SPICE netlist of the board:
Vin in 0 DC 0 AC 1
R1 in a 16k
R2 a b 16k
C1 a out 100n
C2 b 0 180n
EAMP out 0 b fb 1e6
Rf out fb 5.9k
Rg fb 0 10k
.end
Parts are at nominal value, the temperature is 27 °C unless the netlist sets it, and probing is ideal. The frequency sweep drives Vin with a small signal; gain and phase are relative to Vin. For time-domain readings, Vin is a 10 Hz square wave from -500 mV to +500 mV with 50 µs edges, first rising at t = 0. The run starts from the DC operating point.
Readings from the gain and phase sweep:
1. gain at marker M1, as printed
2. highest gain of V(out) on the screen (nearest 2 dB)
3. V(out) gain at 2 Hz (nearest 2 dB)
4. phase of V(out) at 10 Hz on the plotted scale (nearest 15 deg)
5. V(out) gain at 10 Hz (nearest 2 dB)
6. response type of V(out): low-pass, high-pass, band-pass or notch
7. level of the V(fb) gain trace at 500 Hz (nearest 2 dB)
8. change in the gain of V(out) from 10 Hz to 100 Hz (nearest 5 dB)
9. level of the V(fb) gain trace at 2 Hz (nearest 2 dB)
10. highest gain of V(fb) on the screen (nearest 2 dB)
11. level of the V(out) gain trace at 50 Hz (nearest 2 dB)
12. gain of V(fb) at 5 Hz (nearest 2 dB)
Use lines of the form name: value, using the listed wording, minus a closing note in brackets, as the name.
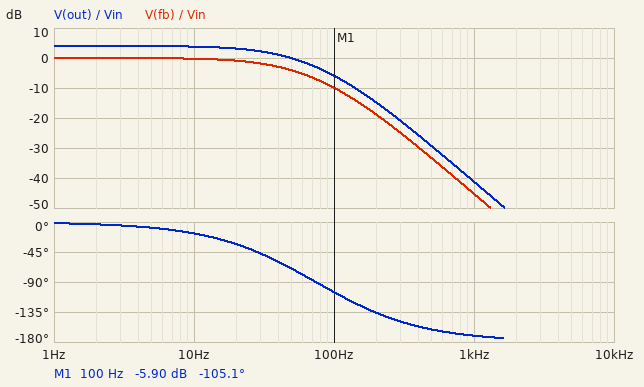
gain at marker M1, as printed: -5.90 dB
highest gain of V(out) on the screen: 4 dB
V(out) gain at 2 Hz: 4 dB
phase of V(out) at 10 Hz on the plotted scale: -15 deg
V(out) gain at 10 Hz: 4 dB
response type of V(out): low-pass, high-pass, band-pass or notch: low-pass
level of the V(fb) gain trace at 500 Hz: -34 dB
change in the gain of V(out) from 10 Hz to 100 Hz: -10 dB
level of the V(fb) gain trace at 2 Hz: 0 dB
highest gain of V(fb) on the screen: 0 dB
level of the V(out) gain trace at 50 Hz: 0 dB
gain of V(fb) at 5 Hz: 0 dB
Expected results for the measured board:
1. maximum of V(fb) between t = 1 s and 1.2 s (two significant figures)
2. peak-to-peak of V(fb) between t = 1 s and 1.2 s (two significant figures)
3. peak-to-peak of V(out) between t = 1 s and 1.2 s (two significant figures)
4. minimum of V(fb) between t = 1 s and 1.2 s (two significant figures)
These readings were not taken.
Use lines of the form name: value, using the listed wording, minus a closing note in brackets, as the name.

maximum of V(fb) between t = 1 s and 1.2 s: 500 mV
peak-to-peak of V(fb) between t = 1 s and 1.2 s: 1.0 V
peak-to-peak of V(out) between t = 1 s and 1.2 s: 1.6 V
minimum of V(fb) between t = 1 s and 1.2 s: -500 mV
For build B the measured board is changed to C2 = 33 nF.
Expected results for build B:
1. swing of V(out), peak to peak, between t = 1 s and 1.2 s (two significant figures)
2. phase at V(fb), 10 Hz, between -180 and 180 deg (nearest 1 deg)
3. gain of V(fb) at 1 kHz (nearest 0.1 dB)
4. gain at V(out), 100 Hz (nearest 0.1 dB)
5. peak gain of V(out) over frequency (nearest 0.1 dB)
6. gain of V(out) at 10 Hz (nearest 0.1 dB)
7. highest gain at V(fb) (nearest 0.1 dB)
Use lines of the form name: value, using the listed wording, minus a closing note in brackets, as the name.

swing of V(out), peak to peak, between t = 1 s and 1.2 s: 4.3 V
phase at V(fb), 10 Hz, between -180 and 180 deg: 0 deg
gain of V(fb) at 1 kHz: -30.2 dB
gain at V(out), 100 Hz: 7.5 dB
peak gain of V(out) over frequency: 22.3 dB
gain of V(out) at 10 Hz: 4.1 dB
highest gain at V(fb): 18.3 dB
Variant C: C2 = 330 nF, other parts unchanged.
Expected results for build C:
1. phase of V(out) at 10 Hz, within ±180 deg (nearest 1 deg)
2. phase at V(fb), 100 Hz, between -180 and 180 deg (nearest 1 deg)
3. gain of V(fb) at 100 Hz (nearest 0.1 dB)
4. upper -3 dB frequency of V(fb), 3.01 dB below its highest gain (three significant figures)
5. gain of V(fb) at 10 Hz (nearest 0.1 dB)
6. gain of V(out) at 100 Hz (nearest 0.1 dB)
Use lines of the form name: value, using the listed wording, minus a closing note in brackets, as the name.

phase of V(out) at 10 Hz, within ±180 deg: -32 deg
phase at V(fb), 100 Hz, between -180 and 180 deg: -111 deg
gain of V(fb) at 100 Hz: -16.2 dB
upper -3 dB frequency of V(fb), 3.01 dB below its highest gain: 18.2 Hz
gain of V(fb) at 10 Hz: -1.1 dB
gain of V(out) at 100 Hz: -12.2 dB
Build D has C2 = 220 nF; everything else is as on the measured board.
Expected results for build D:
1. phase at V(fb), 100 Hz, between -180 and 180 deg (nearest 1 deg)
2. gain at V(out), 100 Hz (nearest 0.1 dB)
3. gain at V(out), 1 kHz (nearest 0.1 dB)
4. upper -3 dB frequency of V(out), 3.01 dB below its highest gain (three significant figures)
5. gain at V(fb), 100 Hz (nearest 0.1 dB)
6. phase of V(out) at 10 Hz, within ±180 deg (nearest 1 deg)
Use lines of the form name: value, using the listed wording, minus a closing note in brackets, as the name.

phase at V(fb), 100 Hz, between -180 and 180 deg: -108 deg
gain at V(out), 100 Hz: -8.1 dB
gain at V(out), 1 kHz: -43.0 dB
upper -3 dB frequency of V(out), 3.01 dB below its highest gain: 30.6 Hz
gain at V(fb), 100 Hz: -12.1 dB
phase of V(out) at 10 Hz, within ±180 deg: -21 deg
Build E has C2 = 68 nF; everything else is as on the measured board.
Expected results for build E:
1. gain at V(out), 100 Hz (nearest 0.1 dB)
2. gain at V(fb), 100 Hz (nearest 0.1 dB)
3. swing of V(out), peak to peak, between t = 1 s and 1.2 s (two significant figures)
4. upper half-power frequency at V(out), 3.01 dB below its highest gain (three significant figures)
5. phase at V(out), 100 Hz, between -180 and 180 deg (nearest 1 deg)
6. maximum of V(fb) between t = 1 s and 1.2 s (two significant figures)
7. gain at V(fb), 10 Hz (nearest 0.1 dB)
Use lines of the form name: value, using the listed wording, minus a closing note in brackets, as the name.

gain at V(out), 100 Hz: 5.6 dB
gain at V(fb), 100 Hz: 1.6 dB
swing of V(out), peak to peak, between t = 1 s and 1.2 s: 2.2 V
upper half-power frequency at V(out), 3.01 dB below its highest gain: 142 Hz
phase at V(out), 100 Hz, between -180 and 180 deg: -68 deg
maximum of V(fb) between t = 1 s and 1.2 s: 690 mV
gain at V(fb), 10 Hz: 0 dB
